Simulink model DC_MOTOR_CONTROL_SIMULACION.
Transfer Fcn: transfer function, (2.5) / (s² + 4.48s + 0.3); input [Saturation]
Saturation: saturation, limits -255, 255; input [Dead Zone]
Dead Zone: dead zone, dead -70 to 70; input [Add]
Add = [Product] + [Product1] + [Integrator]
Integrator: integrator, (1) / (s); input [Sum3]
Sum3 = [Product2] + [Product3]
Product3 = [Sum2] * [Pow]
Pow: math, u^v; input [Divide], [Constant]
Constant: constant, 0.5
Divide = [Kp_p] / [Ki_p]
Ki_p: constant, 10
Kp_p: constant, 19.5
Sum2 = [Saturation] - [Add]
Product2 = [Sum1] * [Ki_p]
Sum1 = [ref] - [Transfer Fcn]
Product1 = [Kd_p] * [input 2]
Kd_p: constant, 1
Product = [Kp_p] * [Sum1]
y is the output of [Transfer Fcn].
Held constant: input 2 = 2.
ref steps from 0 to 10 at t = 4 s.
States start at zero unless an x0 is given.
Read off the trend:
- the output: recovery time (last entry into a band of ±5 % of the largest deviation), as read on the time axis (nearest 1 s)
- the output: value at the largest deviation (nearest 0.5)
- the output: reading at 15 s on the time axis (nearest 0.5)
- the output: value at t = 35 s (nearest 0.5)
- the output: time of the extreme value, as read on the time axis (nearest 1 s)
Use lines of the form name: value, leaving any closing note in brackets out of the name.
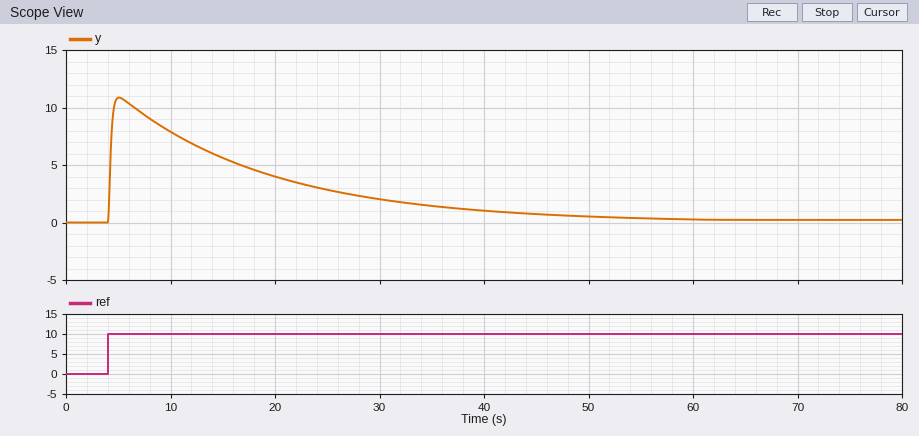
the output: recovery time (last entry into a band of ±5 % of the largest deviation), as read on the time axis: 44 s
the output: value at the largest deviation: 11.0
the output: reading at 15 s on the time axis: 5.5
the output: value at t = 35 s: 1.5
the output: time of the extreme value, as read on the time axis: 5 s
